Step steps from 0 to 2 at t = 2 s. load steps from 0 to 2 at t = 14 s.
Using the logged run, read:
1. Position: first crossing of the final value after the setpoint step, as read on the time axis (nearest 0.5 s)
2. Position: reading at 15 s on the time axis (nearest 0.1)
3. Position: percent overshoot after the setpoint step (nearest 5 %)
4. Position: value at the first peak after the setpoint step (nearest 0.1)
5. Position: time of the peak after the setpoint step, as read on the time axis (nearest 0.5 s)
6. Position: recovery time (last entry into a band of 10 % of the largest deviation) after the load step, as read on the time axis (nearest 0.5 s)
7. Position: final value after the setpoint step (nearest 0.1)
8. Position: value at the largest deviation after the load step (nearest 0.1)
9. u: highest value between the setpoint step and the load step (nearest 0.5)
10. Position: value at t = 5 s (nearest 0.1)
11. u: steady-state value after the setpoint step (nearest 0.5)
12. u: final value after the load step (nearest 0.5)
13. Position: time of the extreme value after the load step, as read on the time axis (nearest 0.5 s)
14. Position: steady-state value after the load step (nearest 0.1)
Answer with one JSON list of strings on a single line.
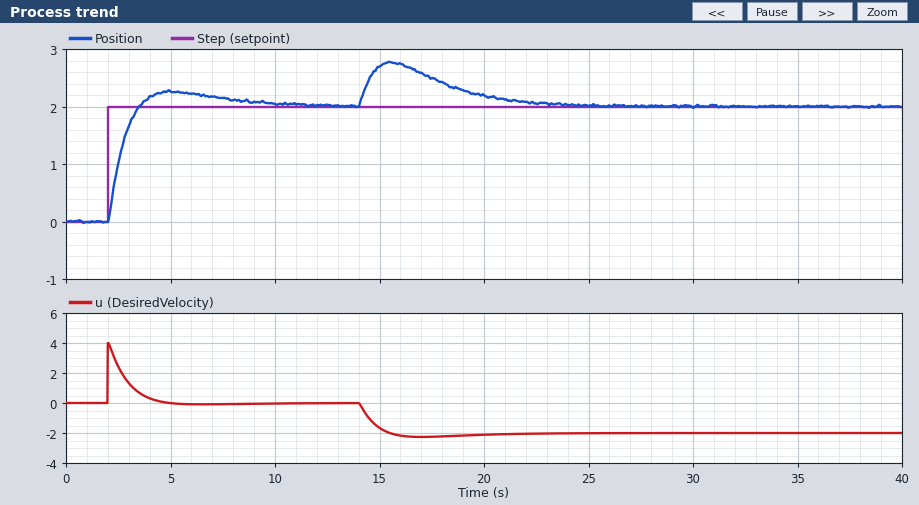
["3.5 s", "2.7", "15 %", "2.3", "5.0 s", "22.0 s", "2.0", "2.8", "4.0", "2.3", "0.0", "-2.0", "15.5 s", "2.0"]
